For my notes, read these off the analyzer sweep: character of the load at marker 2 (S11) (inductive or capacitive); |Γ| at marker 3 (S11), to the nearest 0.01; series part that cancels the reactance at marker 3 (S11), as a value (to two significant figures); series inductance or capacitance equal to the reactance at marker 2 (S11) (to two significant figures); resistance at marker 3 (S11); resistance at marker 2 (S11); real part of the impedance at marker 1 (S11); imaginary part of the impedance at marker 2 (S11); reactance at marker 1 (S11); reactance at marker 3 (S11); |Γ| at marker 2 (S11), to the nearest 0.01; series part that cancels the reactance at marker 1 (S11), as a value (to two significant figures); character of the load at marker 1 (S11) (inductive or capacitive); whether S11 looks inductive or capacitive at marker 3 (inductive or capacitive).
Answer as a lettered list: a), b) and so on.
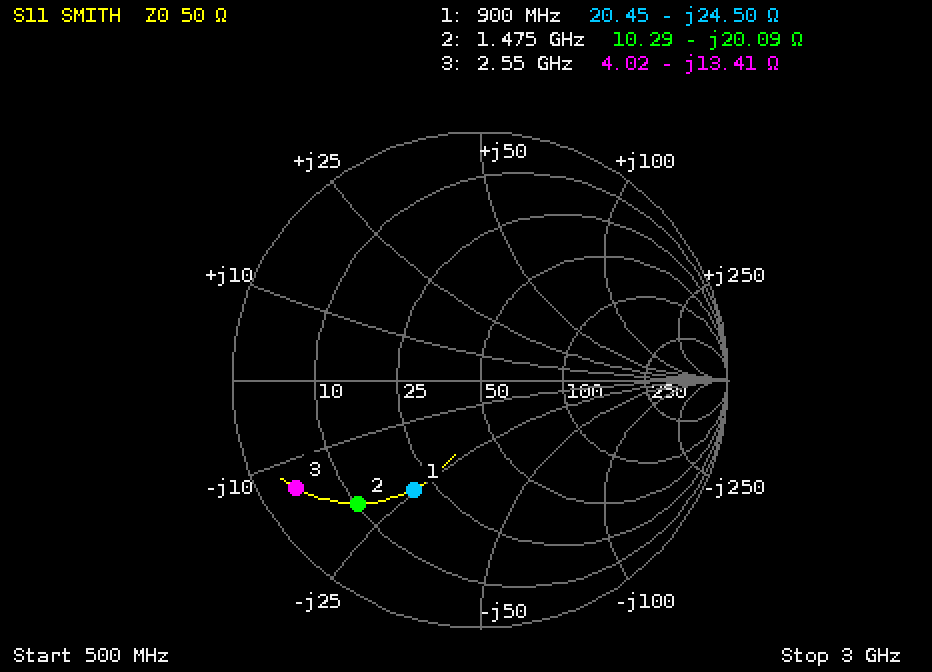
a) capacitive
b) 0.86
c) 840 pH
d) 5.4 pF
e) 4.02 Ω
f) 10.29 Ω
g) 20.45 Ω
h) -20.09 Ω
i) -24.50 Ω
j) -13.41 Ω
k) 0.70
l) 4.3 nH
m) capacitive
n) capacitive
